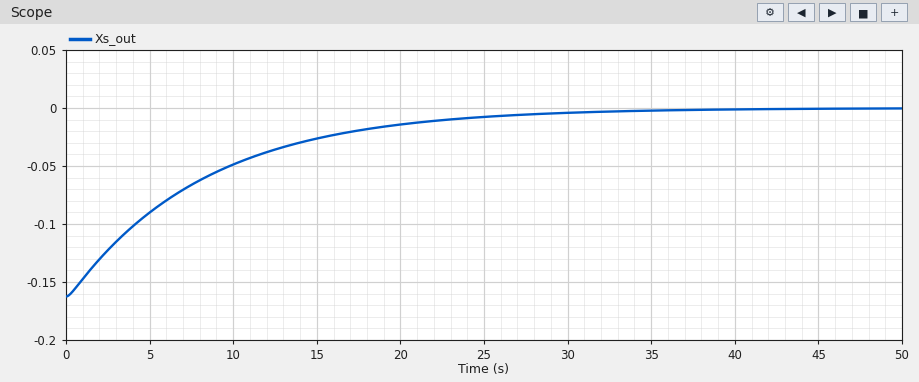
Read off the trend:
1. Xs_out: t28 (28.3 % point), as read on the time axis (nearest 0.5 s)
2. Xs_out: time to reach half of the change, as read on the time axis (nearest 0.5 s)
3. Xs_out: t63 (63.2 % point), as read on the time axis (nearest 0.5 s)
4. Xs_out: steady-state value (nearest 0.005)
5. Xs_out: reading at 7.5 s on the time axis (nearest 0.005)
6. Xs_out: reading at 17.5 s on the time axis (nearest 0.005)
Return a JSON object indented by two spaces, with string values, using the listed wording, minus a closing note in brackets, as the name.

{
  "Xs_out: t28 (28.3 % point), as read on the time axis": "3.0 s",
  "Xs_out: time to reach half of the change, as read on the time axis": "6.0 s",
  "Xs_out: t63 (63.2 % point), as read on the time axis": "8.5 s",
  "Xs_out: steady-state value": "0.000",
  "Xs_out: reading at 7.5 s on the time axis": "-0.065",
  "Xs_out: reading at 17.5 s on the time axis": "-0.020"
}
